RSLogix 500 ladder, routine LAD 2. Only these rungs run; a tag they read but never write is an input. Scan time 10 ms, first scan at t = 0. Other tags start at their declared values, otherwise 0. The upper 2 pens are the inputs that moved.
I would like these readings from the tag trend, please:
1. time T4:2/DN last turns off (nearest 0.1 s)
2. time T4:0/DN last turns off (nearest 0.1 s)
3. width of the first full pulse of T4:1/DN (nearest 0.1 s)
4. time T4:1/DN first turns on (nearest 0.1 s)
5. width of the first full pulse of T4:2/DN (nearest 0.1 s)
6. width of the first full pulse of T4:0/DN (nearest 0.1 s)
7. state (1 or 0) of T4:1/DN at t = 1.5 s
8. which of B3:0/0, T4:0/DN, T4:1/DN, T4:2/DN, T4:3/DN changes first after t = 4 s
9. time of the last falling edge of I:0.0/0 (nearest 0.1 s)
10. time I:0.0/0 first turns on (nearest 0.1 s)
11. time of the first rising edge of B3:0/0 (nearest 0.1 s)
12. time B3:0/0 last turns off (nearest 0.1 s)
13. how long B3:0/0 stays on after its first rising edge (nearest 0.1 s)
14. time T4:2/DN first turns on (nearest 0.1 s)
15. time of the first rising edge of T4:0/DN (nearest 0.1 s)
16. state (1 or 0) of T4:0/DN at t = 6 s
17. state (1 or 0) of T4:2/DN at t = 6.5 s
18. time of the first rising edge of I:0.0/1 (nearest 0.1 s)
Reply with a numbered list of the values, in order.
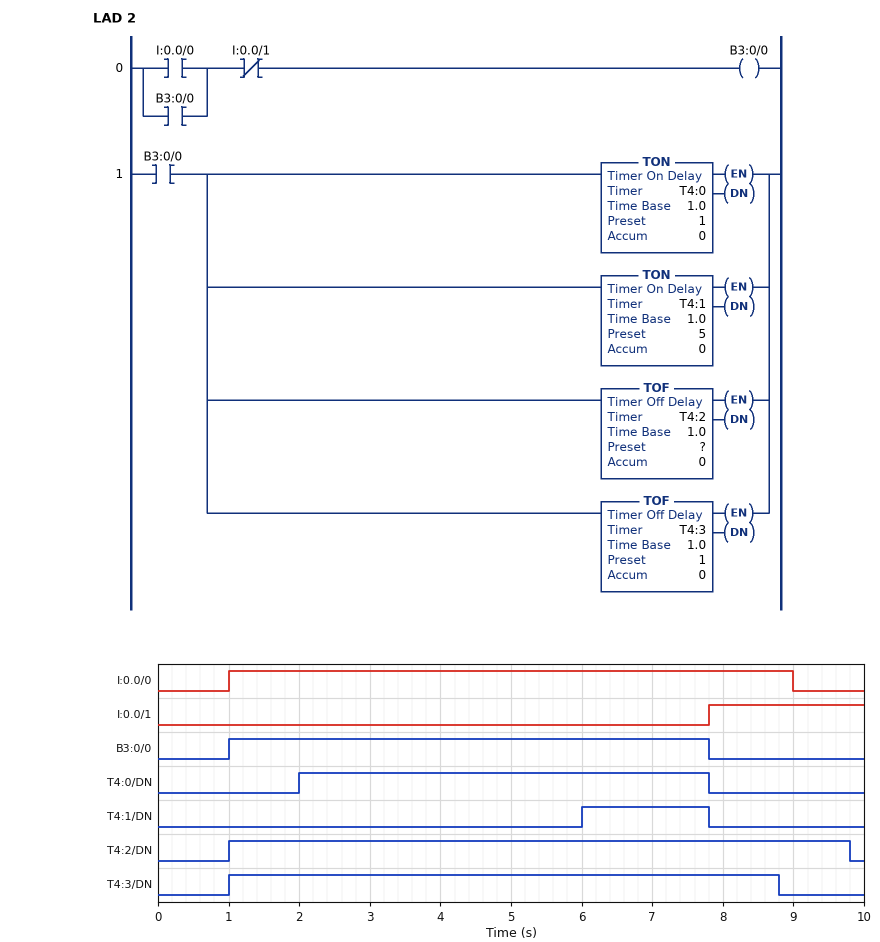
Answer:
1. 9.8 s
2. 7.8 s
3. 1.8 s
4. 6.0 s
5. 8.8 s
6. 5.8 s
7. 0
8. T4:1/DN
9. 9.0 s
10. 1.0 s
11. 1.0 s
12. 7.8 s
13. 6.8 s
14. 1.0 s
15. 2.0 s
16. 1
17. 1
18. 7.8 s
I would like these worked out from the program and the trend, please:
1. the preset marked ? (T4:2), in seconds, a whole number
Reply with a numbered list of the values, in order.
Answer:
1. 2 s
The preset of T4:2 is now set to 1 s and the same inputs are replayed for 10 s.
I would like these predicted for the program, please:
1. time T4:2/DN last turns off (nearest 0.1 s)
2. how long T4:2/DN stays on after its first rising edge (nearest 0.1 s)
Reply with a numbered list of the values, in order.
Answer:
1. 8.8 s
2. 7.8 s
